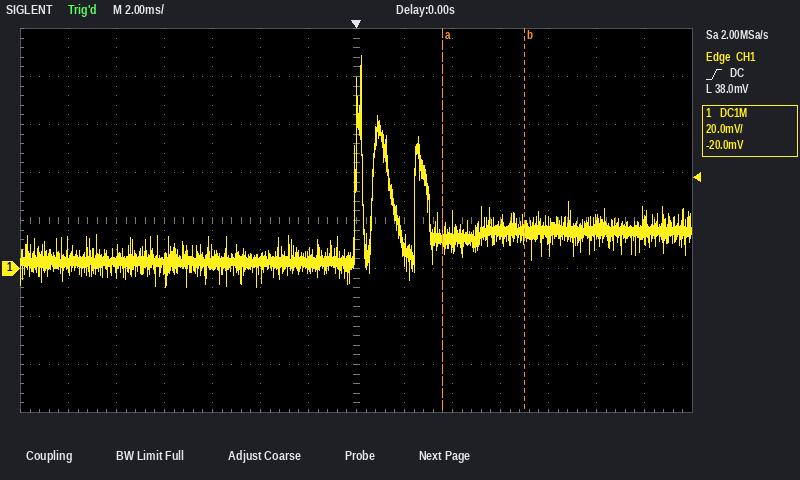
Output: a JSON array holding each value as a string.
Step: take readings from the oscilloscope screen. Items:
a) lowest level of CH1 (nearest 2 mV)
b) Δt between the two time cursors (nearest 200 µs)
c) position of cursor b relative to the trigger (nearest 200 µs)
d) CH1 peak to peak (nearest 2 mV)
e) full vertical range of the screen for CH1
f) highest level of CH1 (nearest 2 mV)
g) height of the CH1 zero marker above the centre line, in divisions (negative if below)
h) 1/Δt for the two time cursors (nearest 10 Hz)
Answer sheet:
["-8 mV", "3.4 ms", "+7.0 ms", "96 mV", "160 mV", "88 mV", "-1.0 div", "290 Hz"]
